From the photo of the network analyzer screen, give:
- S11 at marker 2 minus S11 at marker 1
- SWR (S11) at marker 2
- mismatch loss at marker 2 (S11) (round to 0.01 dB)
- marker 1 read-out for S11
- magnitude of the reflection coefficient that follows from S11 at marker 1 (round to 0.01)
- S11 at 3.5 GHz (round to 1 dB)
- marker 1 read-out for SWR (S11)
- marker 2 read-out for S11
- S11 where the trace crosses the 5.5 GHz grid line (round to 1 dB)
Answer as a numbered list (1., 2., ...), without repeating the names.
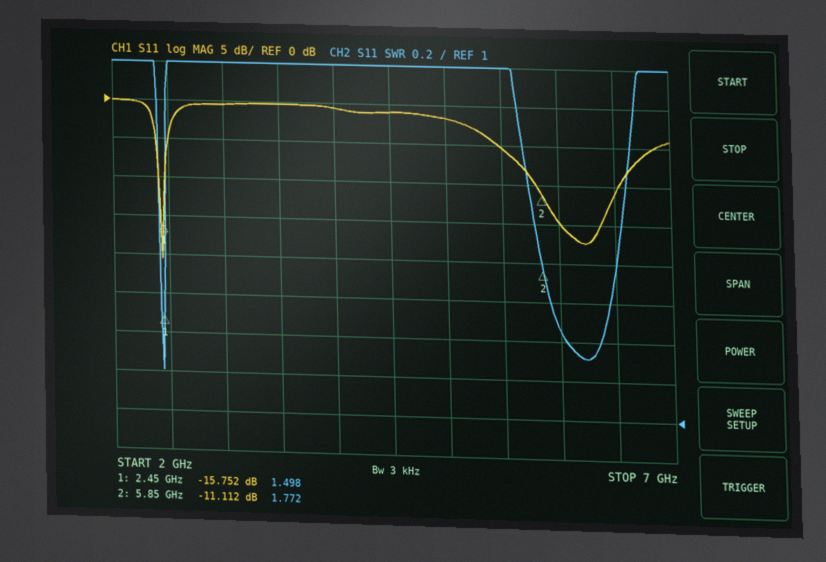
1. 4.640 dB
2. 1.772
3. 0.35 dB
4. -15.752 dB
5. 0.16
6. 0 dB
7. 1.498
8. -11.112 dB
9. -5 dB
